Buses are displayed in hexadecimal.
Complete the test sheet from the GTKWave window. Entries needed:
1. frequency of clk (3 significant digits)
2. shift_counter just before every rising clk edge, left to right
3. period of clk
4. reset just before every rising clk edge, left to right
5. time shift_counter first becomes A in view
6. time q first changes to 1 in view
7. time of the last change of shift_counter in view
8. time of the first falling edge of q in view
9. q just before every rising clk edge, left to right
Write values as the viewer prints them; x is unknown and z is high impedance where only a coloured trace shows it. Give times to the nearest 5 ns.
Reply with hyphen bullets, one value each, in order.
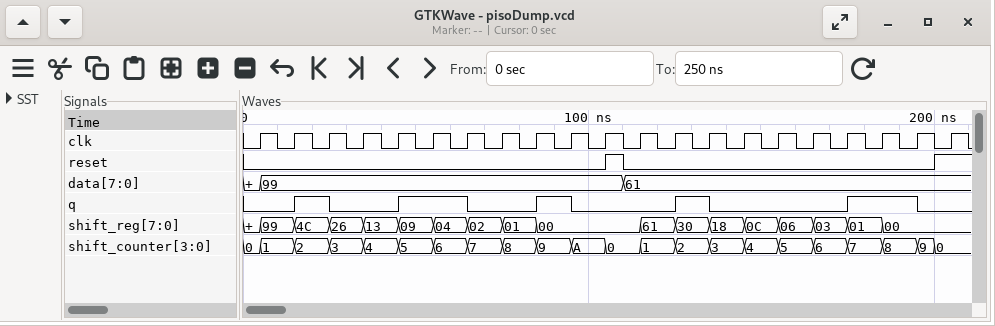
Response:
- 100 MHz
- 0, 1, 2, 3, 4, 5, 6, 7, 8, 9, A, 0, 1, 2, 3, 4, 5, 6, 7, 8, 0
- 10 ns
- 0 0 0 0 0 0 0 0 0 0 0 0 0 0 0 0 0 0 0 0 1
- 95 ns
- 15 ns
- 200 ns
- 25 ns
- 0 0 1 0 0 1 1 0 0 1 0 0 0 1 0 0 0 0 1 1 0
